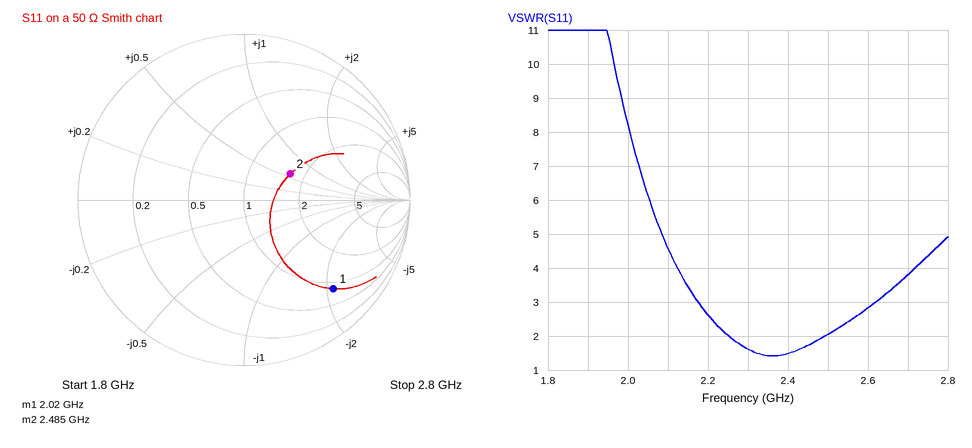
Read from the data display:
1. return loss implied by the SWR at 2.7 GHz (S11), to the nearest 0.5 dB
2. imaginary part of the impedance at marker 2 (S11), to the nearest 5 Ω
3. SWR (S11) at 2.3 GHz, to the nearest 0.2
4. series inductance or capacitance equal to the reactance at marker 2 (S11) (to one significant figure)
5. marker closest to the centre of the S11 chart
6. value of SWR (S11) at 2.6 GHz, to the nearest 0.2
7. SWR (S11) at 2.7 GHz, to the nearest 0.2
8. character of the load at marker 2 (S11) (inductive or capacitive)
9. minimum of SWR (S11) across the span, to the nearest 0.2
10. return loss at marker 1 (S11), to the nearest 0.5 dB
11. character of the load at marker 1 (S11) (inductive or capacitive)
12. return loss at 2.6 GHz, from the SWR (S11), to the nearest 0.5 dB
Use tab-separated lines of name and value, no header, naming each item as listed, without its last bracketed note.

return loss implied by the SWR at 2.7 GHz (S11), to the nearest 0.5 dB	4.5 dB
imaginary part of the impedance at marker 2 (S11), to the nearest 5 Ω	+30 Ω
SWR (S11) at 2.3 GHz, to the nearest 0.2	1.6
series inductance or capacitance equal to the reactance at marker 2 (S11)	2 nH
marker closest to the centre of the S11 chart	marker 2
value of SWR (S11) at 2.6 GHz, to the nearest 0.2	2.8
SWR (S11) at 2.7 GHz, to the nearest 0.2	3.8
character of the load at marker 2 (S11)	inductive
minimum of SWR (S11) across the span, to the nearest 0.2	1.4
return loss at marker 1 (S11), to the nearest 0.5 dB	2.5 dB
character of the load at marker 1 (S11)	capacitive
return loss at 2.6 GHz, from the SWR (S11), to the nearest 0.5 dB	6.5 dB
